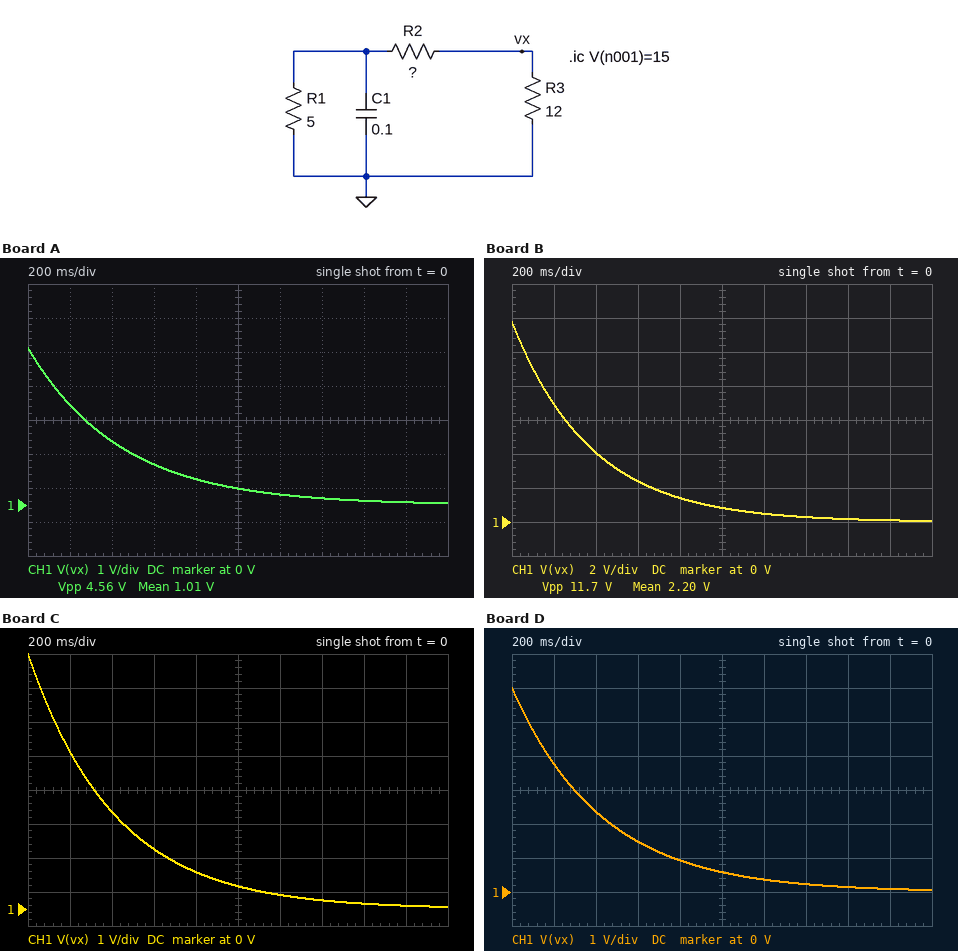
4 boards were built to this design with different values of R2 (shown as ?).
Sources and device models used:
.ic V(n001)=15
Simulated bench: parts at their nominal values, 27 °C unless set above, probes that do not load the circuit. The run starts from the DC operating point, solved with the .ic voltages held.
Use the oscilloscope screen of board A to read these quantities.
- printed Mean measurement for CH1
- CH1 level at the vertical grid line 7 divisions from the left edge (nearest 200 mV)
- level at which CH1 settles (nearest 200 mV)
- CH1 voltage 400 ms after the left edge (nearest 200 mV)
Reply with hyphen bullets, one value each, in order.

- 1.01 V
- 200 mV
- 0 V
- 1.8 V
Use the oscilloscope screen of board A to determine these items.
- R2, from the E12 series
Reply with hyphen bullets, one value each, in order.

- 27 Ω
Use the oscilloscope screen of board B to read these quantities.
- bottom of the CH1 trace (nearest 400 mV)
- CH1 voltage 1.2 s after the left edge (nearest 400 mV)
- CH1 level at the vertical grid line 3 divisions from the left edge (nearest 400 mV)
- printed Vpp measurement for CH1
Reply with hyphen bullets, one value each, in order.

- 0 V
- 400 mV
- 2.4 V
- 11.7 V
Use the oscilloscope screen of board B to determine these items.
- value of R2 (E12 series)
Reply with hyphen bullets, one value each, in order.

- 3.3 Ω
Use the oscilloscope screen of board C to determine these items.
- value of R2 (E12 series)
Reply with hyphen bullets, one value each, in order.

- 12 Ω
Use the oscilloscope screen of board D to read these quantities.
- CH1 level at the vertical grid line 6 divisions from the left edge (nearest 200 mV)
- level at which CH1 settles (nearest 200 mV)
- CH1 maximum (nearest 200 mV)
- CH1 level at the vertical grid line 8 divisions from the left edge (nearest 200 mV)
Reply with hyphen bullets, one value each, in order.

- 400 mV
- 0 V
- 6.0 V
- 200 mV
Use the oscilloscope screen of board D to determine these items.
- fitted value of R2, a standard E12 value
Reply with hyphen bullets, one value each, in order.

- 18 Ω
